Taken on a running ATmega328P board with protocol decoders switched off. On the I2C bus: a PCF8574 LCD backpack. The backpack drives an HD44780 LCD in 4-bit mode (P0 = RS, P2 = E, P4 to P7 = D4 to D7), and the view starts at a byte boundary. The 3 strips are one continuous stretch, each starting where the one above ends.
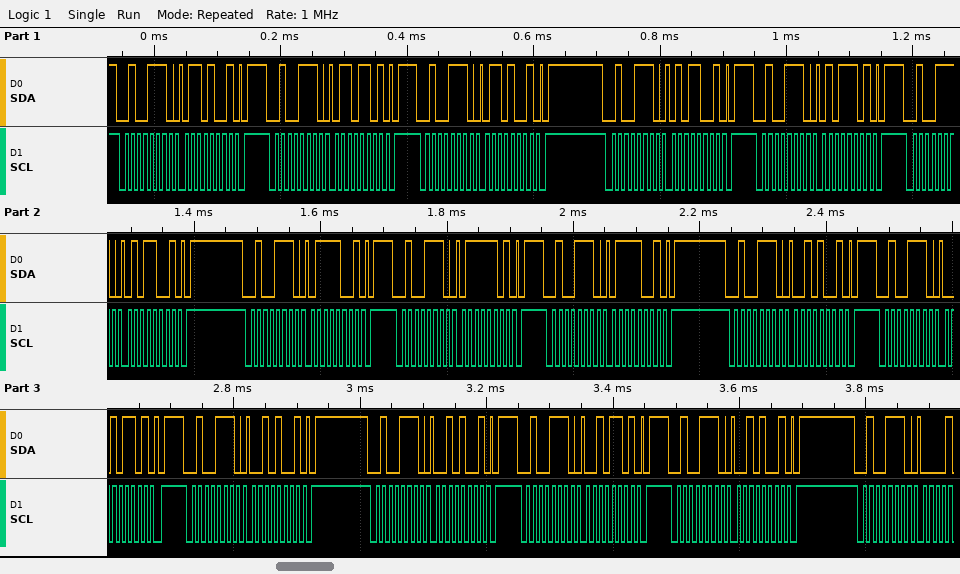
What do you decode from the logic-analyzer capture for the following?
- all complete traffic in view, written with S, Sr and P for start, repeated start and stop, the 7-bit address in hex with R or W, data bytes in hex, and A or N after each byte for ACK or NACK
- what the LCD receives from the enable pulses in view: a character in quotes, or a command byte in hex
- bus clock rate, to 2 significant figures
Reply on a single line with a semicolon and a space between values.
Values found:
S 27W A 69 A P S 27W A 6D A P S 27W A 69 A P S 27W A 59 A P S 27W A 5D A P S 27W A 59 A P S 27W A 79 A P S 27W A 7D A P S 27W A 79 A P S 27W A 29 A P S 27W A 2D A P S 27W A 29 A P S 27W A 29 A P S 27W A 2D A P S 27W A 29 A P S 27W A; 'e' 'r'; 100 kHz
